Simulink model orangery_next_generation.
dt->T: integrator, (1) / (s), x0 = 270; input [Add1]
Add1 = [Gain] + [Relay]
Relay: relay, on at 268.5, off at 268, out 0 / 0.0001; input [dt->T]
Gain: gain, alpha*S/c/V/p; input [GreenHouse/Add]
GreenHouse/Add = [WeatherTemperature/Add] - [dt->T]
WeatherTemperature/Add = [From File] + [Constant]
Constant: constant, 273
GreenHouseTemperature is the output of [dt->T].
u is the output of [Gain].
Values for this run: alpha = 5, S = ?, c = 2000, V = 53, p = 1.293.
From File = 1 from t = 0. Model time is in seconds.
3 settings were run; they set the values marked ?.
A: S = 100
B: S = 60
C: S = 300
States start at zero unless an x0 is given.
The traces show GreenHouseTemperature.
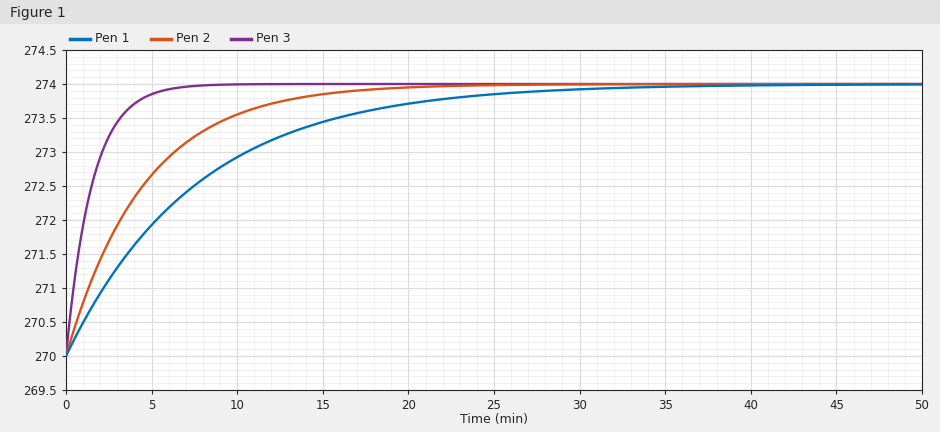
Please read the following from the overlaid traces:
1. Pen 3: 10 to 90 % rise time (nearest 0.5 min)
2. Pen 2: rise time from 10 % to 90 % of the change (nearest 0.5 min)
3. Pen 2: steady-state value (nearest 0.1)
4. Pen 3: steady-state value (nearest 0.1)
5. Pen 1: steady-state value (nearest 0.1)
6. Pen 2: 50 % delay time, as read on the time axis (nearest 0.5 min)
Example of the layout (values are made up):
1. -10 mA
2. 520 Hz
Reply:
1. 3.5 min
2. 10.0 min
3. 274.0
4. 274.0
5. 274.0
6. 3.0 min
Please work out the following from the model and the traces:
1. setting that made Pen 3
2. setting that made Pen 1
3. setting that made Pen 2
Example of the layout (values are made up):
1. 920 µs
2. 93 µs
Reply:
1. C
2. B
3. A
